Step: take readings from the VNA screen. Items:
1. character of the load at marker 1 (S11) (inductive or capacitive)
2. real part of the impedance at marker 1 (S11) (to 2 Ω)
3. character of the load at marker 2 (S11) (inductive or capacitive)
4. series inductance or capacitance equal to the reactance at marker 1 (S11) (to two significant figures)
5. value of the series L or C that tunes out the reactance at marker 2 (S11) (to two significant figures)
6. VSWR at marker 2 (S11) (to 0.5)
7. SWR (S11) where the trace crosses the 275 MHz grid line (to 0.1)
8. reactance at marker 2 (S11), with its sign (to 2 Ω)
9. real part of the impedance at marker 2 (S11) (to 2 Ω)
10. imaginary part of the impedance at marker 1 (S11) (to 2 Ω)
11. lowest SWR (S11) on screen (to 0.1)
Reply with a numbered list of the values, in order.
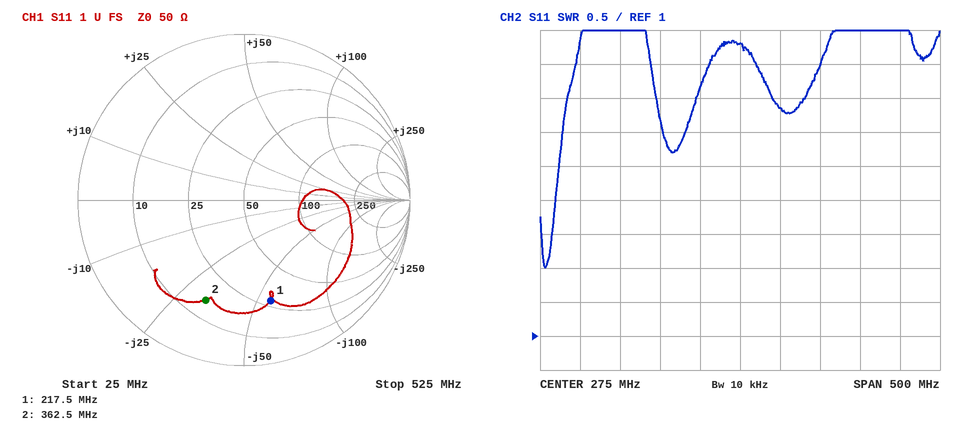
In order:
1. capacitive
2. 28 Ω
3. capacitive
4. 13 pF
5. 14 nH
6. 4.5
7. 5.3
8. -32 Ω
9. 16 Ω
10. -56 Ω
11. 2.0
